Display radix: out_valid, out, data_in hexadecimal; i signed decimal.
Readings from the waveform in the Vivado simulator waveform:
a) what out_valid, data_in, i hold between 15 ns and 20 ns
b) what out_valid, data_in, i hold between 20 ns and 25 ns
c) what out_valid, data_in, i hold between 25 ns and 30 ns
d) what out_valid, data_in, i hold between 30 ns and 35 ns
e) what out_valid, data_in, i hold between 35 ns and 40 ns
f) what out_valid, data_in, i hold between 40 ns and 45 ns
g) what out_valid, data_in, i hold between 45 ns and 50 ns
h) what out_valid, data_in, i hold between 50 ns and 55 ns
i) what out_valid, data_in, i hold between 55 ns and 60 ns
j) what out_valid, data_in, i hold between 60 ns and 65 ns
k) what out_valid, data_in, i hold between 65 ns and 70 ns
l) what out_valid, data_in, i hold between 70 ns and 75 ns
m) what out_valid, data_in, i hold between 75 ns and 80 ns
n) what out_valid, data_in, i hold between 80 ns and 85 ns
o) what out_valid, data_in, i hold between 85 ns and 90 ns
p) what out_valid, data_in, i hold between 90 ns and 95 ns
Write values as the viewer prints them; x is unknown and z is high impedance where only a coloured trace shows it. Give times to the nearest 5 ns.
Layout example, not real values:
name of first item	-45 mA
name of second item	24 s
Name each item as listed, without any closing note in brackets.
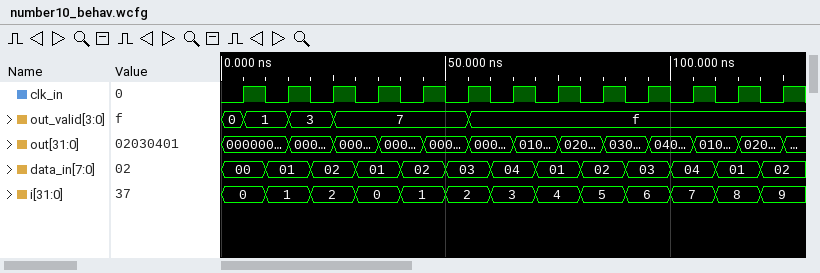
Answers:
what out_valid, data_in, i hold between 15 ns and 20 ns	out_valid=3, data_in=01, i=1
what out_valid, data_in, i hold between 20 ns and 25 ns	out_valid=3, data_in=02, i=2
what out_valid, data_in, i hold between 25 ns and 30 ns	out_valid=7, data_in=02, i=2
what out_valid, data_in, i hold between 30 ns and 35 ns	out_valid=7, data_in=01, i=0
what out_valid, data_in, i hold between 35 ns and 40 ns	out_valid=7, data_in=01, i=0
what out_valid, data_in, i hold between 40 ns and 45 ns	out_valid=7, data_in=02, i=1
what out_valid, data_in, i hold between 45 ns and 50 ns	out_valid=7, data_in=02, i=1
what out_valid, data_in, i hold between 50 ns and 55 ns	out_valid=7, data_in=03, i=2
what out_valid, data_in, i hold between 55 ns and 60 ns	out_valid=f, data_in=03, i=2
what out_valid, data_in, i hold between 60 ns and 65 ns	out_valid=f, data_in=04, i=3
what out_valid, data_in, i hold between 65 ns and 70 ns	out_valid=f, data_in=04, i=3
what out_valid, data_in, i hold between 70 ns and 75 ns	out_valid=f, data_in=01, i=4
what out_valid, data_in, i hold between 75 ns and 80 ns	out_valid=f, data_in=01, i=4
what out_valid, data_in, i hold between 80 ns and 85 ns	out_valid=f, data_in=02, i=5
what out_valid, data_in, i hold between 85 ns and 90 ns	out_valid=f, data_in=02, i=5
what out_valid, data_in, i hold between 90 ns and 95 ns	out_valid=f, data_in=03, i=6
